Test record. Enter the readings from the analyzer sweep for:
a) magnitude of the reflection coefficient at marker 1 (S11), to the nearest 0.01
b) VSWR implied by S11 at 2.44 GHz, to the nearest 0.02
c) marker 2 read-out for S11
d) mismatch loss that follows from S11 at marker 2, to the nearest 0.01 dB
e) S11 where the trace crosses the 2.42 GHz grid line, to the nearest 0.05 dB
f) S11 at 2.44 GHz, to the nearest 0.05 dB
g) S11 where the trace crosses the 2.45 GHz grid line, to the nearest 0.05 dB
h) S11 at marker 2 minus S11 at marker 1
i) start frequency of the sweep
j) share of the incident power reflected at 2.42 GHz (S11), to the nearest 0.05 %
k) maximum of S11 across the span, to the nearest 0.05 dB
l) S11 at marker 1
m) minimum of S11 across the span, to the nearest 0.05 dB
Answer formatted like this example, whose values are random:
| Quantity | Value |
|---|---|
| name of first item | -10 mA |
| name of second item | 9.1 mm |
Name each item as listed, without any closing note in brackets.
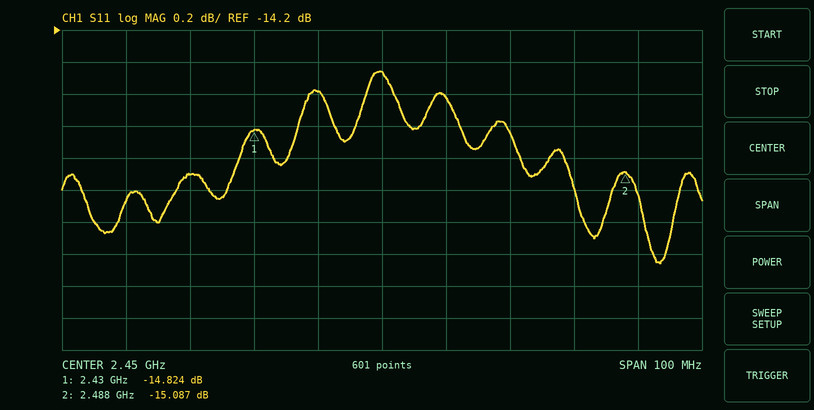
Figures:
| Quantity | Value |
|---|---|
| magnitude of the reflection coefficient at marker 1 (S11), to the nearest 0.01 | 0.18 |
| VSWR implied by S11 at 2.44 GHz, to the nearest 0.02 | 1.46 |
| marker 2 read-out for S11 | -15.087 dB |
| mismatch loss that follows from S11 at marker 2, to the nearest 0.01 dB | 0.14 dB |
| S11 where the trace crosses the 2.42 GHz grid line, to the nearest 0.05 dB | -15.10 dB |
| S11 at 2.44 GHz, to the nearest 0.05 dB | -14.60 dB |
| S11 where the trace crosses the 2.45 GHz grid line, to the nearest 0.05 dB | -14.45 dB |
| S11 at marker 2 minus S11 at marker 1 | -0.263 dB |
| start frequency of the sweep | 2.4 GHz |
| share of the incident power reflected at 2.42 GHz (S11), to the nearest 0.05 % | 3.10 % |
| maximum of S11 across the span, to the nearest 0.05 dB | -14.45 dB |
| S11 at marker 1 | -14.824 dB |
| minimum of S11 across the span, to the nearest 0.05 dB | -15.65 dB |
